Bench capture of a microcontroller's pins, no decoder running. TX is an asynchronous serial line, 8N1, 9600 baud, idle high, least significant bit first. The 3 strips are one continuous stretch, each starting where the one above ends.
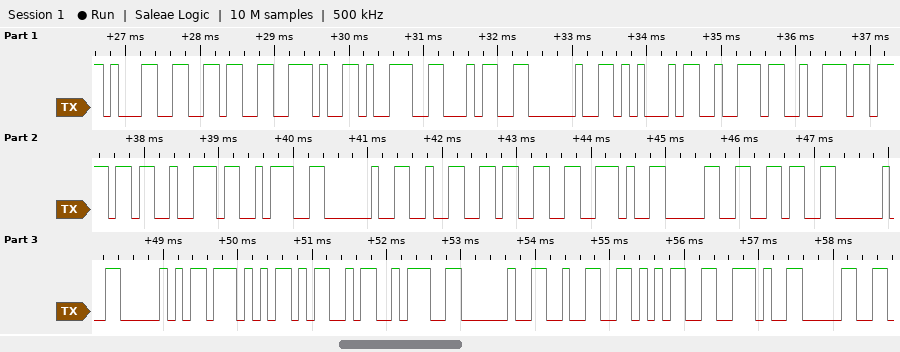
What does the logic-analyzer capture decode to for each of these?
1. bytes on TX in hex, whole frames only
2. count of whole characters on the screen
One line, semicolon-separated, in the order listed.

31 36 2E 39 34 20 45 72 72 6F 72 3A 20 32 33 2E 30 36 20 50 57 4D 3A 20 32 35 2E 30; 28
